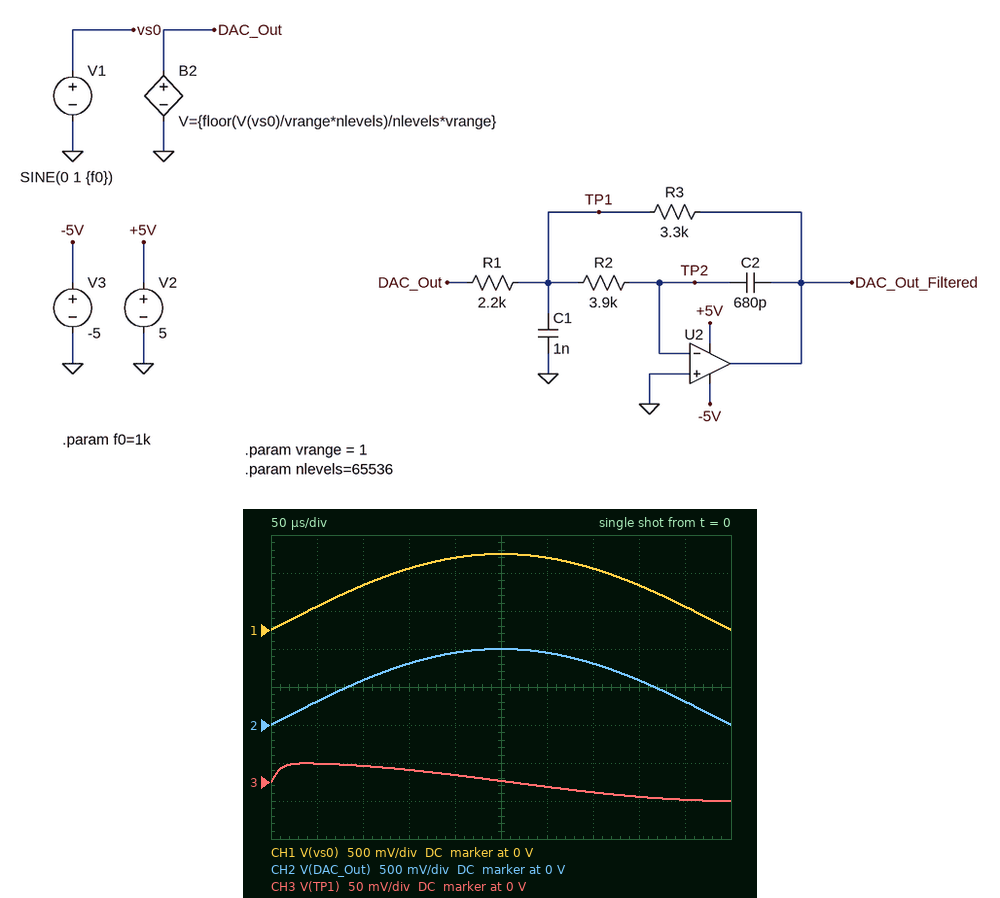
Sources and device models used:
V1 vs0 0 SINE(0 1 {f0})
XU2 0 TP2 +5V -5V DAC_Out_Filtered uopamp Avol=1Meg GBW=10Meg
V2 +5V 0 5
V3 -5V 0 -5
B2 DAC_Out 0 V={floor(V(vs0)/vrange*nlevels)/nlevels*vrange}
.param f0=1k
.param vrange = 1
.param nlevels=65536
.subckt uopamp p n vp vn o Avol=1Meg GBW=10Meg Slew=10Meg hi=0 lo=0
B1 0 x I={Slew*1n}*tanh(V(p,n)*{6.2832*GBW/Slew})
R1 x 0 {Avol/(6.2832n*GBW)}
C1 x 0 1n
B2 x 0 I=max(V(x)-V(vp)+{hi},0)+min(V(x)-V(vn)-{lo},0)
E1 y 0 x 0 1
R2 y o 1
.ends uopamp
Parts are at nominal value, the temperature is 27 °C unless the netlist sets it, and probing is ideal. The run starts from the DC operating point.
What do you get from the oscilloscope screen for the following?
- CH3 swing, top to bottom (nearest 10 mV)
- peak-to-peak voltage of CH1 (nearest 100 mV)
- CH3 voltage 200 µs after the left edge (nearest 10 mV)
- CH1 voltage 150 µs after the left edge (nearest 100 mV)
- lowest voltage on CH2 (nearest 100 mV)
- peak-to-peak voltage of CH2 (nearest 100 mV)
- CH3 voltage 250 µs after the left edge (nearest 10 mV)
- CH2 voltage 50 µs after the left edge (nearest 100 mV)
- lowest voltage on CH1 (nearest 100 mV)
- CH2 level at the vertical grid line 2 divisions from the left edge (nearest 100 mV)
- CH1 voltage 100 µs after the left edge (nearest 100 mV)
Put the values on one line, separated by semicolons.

50 mV; 1.0 V; 10 mV; 800 mV; 0 V; 1.0 V; 0 V; 300 mV; 0 V; 600 mV; 600 mV
